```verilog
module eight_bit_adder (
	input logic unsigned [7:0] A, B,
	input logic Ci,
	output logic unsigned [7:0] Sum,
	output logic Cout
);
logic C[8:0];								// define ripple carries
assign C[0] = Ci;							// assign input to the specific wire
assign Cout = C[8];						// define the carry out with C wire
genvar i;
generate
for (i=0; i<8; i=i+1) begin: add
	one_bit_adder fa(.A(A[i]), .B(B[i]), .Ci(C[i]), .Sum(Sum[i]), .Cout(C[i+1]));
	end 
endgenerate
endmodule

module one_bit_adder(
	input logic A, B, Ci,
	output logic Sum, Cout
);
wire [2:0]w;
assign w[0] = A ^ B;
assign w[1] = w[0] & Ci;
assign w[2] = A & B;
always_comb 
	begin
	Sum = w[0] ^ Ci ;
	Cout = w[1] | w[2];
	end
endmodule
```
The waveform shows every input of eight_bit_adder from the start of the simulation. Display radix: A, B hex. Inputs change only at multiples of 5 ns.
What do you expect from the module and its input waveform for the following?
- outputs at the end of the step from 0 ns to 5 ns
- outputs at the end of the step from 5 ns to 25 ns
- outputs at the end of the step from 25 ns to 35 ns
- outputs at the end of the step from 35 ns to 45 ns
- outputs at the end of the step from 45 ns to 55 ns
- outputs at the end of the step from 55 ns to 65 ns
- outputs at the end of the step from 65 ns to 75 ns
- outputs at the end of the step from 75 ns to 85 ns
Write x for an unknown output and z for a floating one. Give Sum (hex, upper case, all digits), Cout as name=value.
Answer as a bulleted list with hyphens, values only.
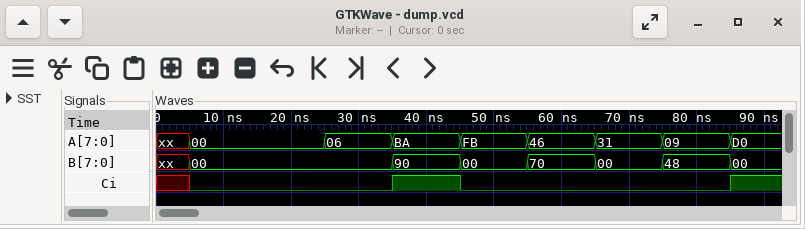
- Sum=x, Cout=x
- Sum=00, Cout=0
- Sum=06, Cout=0
- Sum=4B, Cout=1
- Sum=FB, Cout=0
- Sum=B6, Cout=0
- Sum=31, Cout=0
- Sum=51, Cout=0
